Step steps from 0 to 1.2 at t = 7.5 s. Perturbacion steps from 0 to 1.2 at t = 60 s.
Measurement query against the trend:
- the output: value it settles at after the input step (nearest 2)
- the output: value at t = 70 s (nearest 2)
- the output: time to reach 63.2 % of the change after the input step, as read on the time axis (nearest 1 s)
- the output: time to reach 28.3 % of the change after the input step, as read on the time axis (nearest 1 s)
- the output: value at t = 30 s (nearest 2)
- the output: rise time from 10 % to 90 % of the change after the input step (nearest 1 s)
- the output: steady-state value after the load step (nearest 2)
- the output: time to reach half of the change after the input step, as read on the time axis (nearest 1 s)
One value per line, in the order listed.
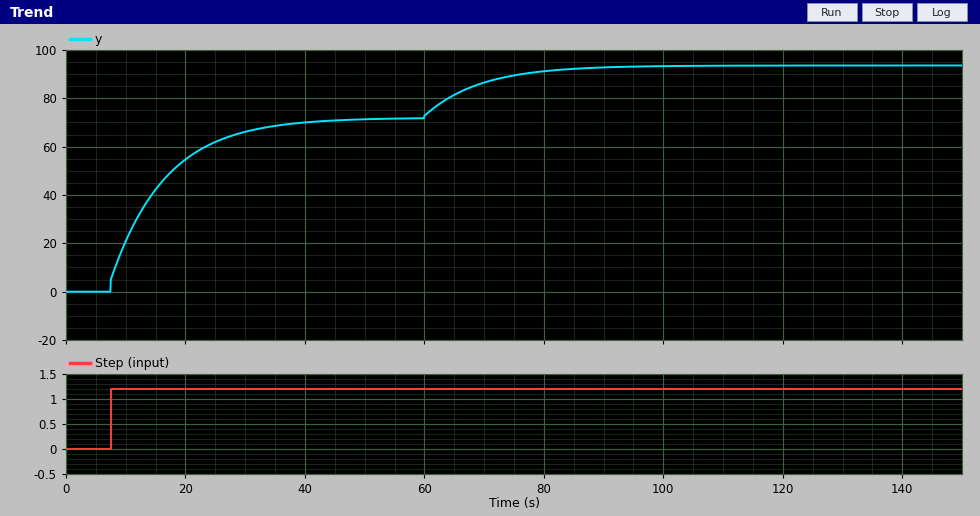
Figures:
72
86
16 s
10 s
66
20 s
94
13 s
